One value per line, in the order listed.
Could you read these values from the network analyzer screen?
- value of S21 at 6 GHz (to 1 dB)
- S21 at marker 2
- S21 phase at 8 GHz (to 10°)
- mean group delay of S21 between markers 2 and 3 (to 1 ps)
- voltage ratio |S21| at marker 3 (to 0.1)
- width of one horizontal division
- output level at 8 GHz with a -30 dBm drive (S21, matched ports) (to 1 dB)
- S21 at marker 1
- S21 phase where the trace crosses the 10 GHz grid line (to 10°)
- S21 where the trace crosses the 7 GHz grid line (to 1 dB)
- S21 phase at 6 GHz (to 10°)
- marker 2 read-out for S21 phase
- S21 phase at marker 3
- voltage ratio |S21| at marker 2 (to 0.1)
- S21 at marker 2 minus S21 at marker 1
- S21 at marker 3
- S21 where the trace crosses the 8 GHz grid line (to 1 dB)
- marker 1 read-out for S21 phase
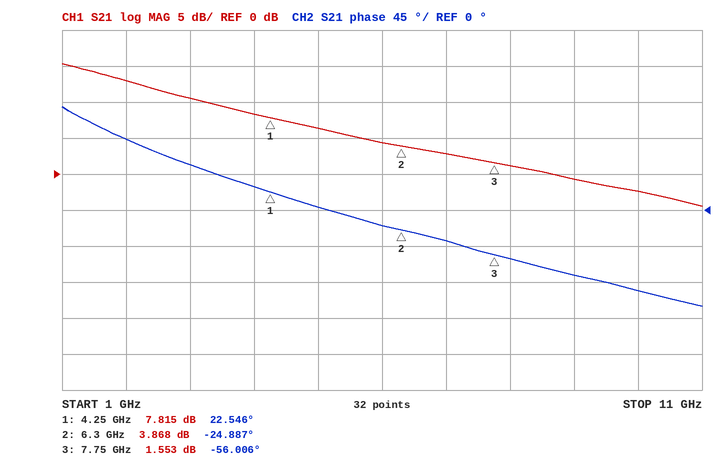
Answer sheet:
4 dB
3.868 dB
-60°
60 ps
1.2
1 GHz
-29 dBm
7.815 dB
-100°
3 dB
-20°
-24.887°
-56.006°
1.6
-3.947 dB
1.553 dB
1 dB
22.546°
